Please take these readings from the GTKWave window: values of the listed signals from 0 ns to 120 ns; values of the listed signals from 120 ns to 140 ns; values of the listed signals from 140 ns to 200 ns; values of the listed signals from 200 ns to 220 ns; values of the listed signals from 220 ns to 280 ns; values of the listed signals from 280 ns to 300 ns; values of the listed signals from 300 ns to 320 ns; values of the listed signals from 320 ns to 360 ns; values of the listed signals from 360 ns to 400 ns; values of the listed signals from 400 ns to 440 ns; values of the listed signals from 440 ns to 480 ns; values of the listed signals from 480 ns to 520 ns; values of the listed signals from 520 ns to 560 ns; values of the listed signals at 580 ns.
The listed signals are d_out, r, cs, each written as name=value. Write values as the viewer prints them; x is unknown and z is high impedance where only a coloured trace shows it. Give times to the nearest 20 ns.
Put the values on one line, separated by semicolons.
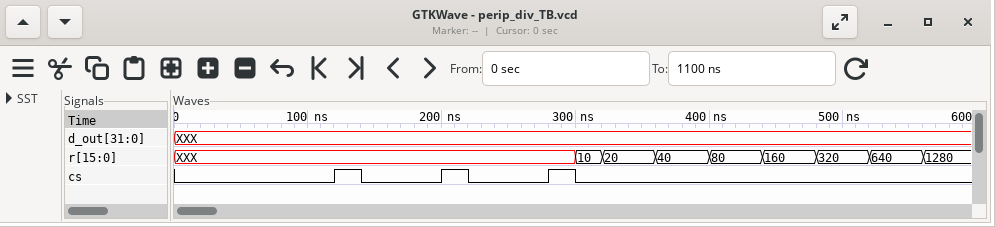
d_out=XXX, r=XXX, cs=0; d_out=XXX, r=XXX, cs=1; d_out=XXX, r=XXX, cs=0; d_out=XXX, r=XXX, cs=1; d_out=XXX, r=XXX, cs=0; d_out=XXX, r=XXX, cs=1; d_out=XXX, r=10, cs=0; d_out=XXX, r=20, cs=0; d_out=XXX, r=40, cs=0; d_out=XXX, r=80, cs=0; d_out=XXX, r=160, cs=0; d_out=XXX, r=320, cs=0; d_out=XXX, r=640, cs=0; d_out=XXX, r=1280, cs=0
